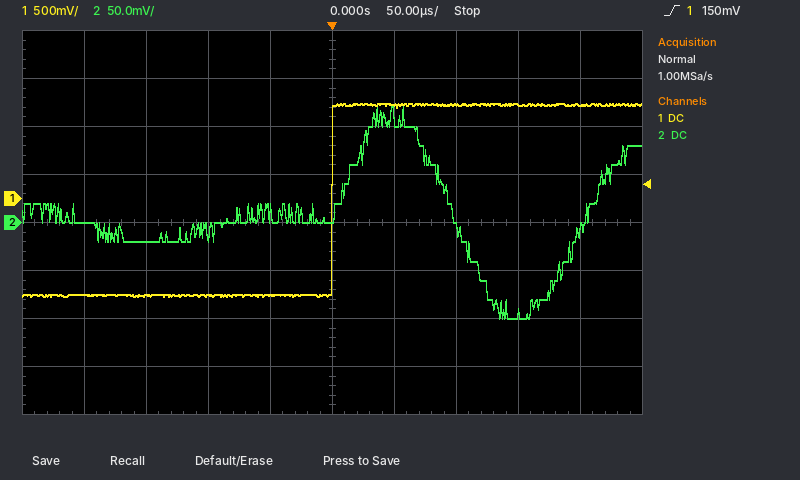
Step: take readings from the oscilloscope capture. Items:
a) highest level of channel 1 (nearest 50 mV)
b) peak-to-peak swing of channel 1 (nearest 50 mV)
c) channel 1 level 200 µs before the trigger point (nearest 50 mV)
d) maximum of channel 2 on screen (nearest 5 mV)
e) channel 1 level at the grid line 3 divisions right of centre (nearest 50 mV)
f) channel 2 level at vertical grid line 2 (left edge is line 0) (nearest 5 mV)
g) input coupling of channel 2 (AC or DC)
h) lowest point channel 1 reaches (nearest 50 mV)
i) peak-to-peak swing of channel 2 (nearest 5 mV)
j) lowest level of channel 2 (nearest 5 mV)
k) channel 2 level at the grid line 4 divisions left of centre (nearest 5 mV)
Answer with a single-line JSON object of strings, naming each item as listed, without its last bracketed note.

{"highest level of channel 1": "1.00 V", "peak-to-peak swing of channel 1": "2.00 V", "channel 1 level 200 µs before the trigger point": "-1.00 V", "maximum of channel 2 on screen": "120 mV", "channel 1 level at the grid line 3 divisions right of centre": "1.00 V", "channel 2 level at vertical grid line 2 (left edge is line 0)": "-20 mV", "input coupling of channel 2": "DC", "lowest point channel 1 reaches": "-1.00 V", "peak-to-peak swing of channel 2": "220 mV", "lowest level of channel 2": "-100 mV", "channel 2 level at the grid line 4 divisions left of centre": "0 mV"}
